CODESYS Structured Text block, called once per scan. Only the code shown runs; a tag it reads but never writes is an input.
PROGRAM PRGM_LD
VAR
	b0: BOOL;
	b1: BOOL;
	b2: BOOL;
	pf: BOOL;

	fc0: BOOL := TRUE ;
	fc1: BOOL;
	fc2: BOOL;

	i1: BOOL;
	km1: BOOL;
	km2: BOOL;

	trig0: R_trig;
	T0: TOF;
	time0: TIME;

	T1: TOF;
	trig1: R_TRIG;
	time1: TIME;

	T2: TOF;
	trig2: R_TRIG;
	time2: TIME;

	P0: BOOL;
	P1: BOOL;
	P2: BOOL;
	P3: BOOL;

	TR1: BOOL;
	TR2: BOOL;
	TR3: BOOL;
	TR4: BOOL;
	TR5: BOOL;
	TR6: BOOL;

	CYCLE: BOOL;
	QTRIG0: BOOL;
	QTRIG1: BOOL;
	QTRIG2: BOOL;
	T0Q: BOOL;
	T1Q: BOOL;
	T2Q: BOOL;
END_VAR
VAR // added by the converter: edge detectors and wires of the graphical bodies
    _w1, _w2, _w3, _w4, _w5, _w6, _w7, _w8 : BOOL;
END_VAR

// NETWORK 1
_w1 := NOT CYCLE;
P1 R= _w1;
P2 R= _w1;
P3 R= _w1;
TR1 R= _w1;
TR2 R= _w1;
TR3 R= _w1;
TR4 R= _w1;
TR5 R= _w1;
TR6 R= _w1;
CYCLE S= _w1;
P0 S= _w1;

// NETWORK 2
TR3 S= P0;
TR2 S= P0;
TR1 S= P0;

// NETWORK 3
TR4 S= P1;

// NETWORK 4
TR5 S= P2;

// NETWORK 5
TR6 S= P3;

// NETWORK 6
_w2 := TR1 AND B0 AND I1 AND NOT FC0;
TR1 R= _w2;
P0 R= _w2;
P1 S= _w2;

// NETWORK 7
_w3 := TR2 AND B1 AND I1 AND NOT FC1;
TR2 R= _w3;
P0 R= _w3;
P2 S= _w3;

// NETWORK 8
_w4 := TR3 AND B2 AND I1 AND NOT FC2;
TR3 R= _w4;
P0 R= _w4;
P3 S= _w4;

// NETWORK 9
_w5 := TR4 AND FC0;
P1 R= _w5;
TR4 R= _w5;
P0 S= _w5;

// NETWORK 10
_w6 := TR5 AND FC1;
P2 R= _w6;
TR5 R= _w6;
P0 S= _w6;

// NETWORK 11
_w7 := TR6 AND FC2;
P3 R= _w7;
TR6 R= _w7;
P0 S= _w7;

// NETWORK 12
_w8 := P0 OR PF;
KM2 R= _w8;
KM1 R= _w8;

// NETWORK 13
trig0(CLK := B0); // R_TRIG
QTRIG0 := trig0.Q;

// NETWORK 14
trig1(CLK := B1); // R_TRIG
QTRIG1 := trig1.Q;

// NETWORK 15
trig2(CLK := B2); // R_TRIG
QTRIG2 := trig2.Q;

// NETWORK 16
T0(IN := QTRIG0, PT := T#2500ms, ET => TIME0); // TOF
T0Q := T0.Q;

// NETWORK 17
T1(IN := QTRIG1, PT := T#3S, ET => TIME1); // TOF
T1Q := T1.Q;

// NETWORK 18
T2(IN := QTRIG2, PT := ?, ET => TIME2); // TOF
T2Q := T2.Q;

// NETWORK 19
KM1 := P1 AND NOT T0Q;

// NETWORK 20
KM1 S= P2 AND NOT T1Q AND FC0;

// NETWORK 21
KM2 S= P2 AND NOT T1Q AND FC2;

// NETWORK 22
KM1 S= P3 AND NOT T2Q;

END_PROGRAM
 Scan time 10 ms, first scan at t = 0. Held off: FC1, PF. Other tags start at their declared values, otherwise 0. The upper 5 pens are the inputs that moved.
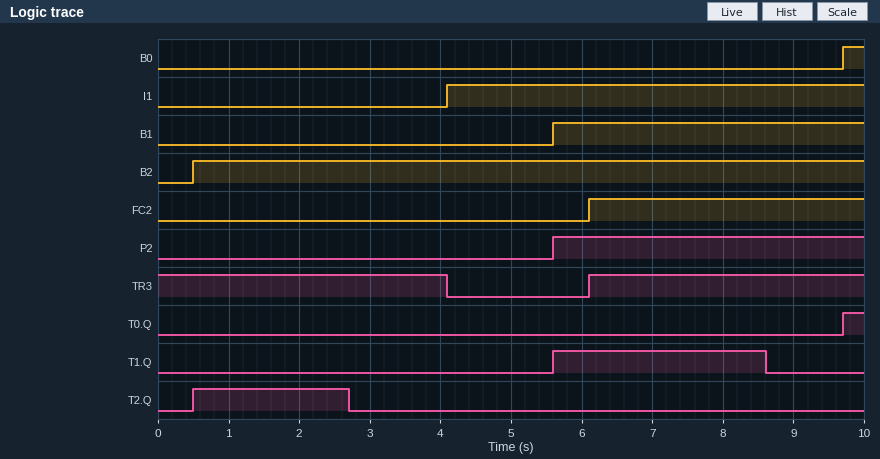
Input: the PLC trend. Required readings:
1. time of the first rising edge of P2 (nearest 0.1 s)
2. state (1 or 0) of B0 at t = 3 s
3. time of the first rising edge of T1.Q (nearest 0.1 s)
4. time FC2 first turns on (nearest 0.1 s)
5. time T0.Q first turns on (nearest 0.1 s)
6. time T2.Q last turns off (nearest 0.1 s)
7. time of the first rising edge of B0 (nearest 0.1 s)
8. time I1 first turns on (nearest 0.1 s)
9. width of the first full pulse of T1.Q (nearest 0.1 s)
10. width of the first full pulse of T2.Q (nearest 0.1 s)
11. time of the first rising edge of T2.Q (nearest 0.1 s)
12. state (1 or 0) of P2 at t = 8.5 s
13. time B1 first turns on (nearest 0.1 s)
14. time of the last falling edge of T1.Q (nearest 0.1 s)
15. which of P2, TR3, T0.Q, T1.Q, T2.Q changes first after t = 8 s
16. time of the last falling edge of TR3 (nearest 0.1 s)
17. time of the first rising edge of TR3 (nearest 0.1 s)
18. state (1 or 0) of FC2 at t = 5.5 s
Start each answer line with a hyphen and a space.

- 5.6 s
- 0
- 5.6 s
- 6.1 s
- 9.7 s
- 2.7 s
- 9.7 s
- 4.1 s
- 3.0 s
- 2.2 s
- 0.5 s
- 1
- 5.6 s
- 8.6 s
- T1.Q
- 4.1 s
- 6.1 s
- 0
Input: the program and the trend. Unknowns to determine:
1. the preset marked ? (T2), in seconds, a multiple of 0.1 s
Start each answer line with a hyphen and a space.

- 2.2 s
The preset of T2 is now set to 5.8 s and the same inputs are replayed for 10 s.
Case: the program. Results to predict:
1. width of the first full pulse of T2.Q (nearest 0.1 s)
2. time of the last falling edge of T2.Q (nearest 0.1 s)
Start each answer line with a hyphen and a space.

- 5.8 s
- 6.3 s
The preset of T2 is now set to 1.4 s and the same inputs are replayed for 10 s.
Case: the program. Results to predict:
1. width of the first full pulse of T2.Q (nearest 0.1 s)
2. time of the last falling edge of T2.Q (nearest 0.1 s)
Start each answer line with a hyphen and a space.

- 1.4 s
- 1.9 s
